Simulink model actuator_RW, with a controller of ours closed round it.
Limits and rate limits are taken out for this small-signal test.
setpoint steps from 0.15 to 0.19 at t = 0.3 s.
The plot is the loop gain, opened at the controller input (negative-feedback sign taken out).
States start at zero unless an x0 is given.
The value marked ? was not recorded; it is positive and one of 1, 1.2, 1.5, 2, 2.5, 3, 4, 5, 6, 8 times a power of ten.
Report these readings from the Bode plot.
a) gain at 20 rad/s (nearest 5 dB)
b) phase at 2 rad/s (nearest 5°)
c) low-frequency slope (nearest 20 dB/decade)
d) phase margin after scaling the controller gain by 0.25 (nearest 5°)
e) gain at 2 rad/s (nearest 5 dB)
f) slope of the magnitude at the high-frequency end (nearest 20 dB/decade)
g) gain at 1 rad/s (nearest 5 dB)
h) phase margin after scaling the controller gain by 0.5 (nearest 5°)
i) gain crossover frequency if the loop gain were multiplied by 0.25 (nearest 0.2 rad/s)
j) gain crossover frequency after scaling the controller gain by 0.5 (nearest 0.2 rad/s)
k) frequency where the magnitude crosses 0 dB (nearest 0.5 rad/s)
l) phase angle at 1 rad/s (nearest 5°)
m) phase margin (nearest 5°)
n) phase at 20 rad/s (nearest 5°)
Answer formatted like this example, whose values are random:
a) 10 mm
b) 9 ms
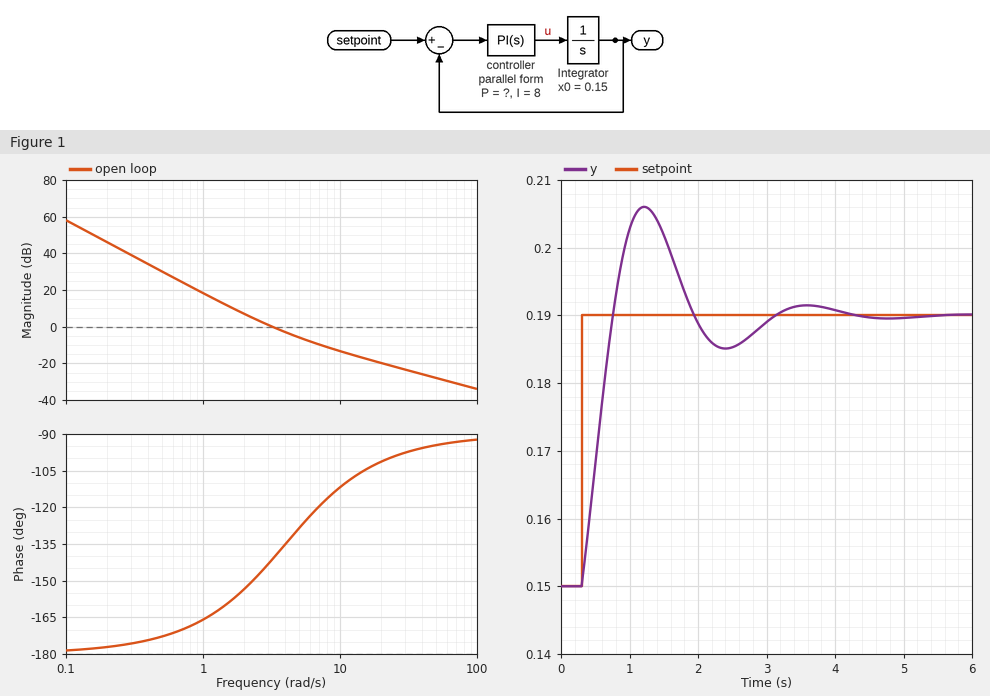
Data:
a) -20 dB
b) -155°
c) -40 dB/decade
d) 20°
e) 5 dB
f) -20 dB/decade
g) 20 dB
h) 30°
i) 1.4 rad/s
j) 2.2 rad/s
k) 3.0 rad/s
l) -165°
m) 40°
n) -100°
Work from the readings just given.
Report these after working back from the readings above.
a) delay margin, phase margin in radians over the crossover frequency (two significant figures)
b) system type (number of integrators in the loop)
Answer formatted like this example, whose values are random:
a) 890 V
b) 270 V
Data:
a) 0.23 s
b) 2
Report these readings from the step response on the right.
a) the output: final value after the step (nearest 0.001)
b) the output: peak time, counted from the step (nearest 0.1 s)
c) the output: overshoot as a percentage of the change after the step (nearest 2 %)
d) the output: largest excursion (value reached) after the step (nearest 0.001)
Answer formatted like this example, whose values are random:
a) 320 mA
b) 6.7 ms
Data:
a) 0.190
b) 0.9 s
c) 40 %
d) 0.206
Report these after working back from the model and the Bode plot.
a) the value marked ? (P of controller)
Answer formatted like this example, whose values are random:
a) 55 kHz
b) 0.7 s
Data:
a) 2
